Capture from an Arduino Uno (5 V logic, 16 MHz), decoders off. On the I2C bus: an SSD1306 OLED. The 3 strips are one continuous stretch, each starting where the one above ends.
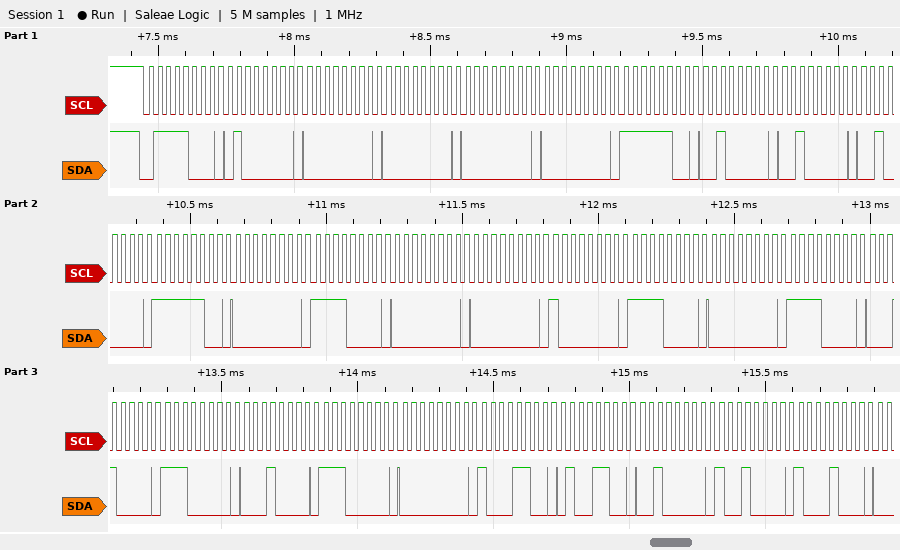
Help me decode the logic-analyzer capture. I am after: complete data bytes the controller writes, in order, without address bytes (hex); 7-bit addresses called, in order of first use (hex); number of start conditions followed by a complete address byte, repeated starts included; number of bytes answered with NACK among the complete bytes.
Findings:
40 00 00 00 00 FC 20 20 20 FC 00 F0 00 00 80 F0 00 F0 10 E0 10 E0 00 8C 4C 20 90 88
0x3C
1
0
